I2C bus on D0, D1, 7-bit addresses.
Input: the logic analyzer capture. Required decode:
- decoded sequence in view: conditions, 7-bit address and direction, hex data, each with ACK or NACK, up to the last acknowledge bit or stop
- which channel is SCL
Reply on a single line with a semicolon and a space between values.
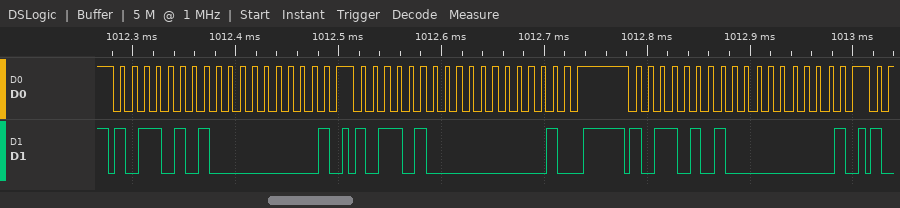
start, address 5A read ACK, 00 NACK, stop, start, address 5A write ACK, 01 ACK, stop, start, address 5A read ACK, 00 NACK, stop; D0
